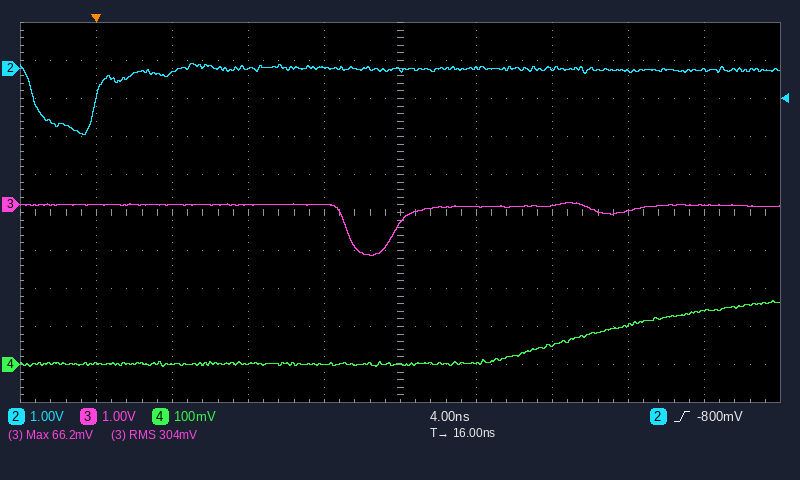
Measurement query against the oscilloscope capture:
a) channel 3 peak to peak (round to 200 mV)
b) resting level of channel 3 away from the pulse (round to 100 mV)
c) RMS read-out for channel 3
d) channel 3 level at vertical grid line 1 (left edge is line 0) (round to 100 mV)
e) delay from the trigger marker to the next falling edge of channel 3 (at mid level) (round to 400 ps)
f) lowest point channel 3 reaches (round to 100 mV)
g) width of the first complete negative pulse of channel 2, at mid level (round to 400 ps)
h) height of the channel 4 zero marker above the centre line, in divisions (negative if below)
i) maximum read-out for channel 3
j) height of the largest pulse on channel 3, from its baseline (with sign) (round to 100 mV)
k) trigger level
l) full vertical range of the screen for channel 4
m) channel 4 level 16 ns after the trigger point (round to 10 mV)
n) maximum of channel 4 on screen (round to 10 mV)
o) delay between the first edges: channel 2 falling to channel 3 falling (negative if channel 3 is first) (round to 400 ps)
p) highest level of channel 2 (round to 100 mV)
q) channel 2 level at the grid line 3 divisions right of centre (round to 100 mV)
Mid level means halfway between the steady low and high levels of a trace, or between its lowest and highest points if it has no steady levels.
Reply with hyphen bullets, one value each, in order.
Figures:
- 1.4 V
- 0.0 V
- 304 mV
- 0.0 V
- 13.2 ns
- -1.3 V
- 3.2 ns
- -4.0 div
- 66.2 mV
- -1.3 V
- -800 mV
- 1 V
- 0 mV
- 170 mV
- +16.4 ns
- 100 mV
- -100 mV
